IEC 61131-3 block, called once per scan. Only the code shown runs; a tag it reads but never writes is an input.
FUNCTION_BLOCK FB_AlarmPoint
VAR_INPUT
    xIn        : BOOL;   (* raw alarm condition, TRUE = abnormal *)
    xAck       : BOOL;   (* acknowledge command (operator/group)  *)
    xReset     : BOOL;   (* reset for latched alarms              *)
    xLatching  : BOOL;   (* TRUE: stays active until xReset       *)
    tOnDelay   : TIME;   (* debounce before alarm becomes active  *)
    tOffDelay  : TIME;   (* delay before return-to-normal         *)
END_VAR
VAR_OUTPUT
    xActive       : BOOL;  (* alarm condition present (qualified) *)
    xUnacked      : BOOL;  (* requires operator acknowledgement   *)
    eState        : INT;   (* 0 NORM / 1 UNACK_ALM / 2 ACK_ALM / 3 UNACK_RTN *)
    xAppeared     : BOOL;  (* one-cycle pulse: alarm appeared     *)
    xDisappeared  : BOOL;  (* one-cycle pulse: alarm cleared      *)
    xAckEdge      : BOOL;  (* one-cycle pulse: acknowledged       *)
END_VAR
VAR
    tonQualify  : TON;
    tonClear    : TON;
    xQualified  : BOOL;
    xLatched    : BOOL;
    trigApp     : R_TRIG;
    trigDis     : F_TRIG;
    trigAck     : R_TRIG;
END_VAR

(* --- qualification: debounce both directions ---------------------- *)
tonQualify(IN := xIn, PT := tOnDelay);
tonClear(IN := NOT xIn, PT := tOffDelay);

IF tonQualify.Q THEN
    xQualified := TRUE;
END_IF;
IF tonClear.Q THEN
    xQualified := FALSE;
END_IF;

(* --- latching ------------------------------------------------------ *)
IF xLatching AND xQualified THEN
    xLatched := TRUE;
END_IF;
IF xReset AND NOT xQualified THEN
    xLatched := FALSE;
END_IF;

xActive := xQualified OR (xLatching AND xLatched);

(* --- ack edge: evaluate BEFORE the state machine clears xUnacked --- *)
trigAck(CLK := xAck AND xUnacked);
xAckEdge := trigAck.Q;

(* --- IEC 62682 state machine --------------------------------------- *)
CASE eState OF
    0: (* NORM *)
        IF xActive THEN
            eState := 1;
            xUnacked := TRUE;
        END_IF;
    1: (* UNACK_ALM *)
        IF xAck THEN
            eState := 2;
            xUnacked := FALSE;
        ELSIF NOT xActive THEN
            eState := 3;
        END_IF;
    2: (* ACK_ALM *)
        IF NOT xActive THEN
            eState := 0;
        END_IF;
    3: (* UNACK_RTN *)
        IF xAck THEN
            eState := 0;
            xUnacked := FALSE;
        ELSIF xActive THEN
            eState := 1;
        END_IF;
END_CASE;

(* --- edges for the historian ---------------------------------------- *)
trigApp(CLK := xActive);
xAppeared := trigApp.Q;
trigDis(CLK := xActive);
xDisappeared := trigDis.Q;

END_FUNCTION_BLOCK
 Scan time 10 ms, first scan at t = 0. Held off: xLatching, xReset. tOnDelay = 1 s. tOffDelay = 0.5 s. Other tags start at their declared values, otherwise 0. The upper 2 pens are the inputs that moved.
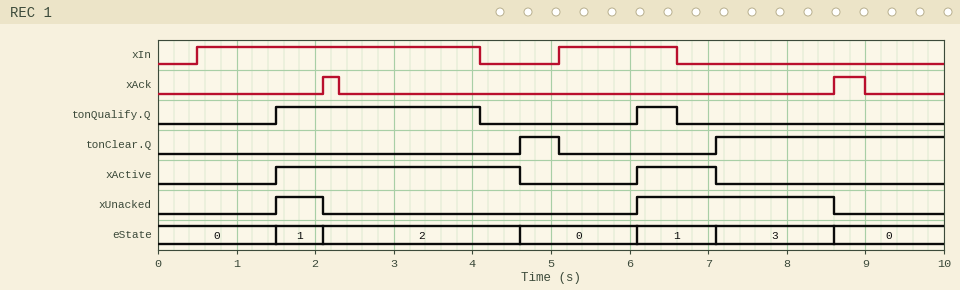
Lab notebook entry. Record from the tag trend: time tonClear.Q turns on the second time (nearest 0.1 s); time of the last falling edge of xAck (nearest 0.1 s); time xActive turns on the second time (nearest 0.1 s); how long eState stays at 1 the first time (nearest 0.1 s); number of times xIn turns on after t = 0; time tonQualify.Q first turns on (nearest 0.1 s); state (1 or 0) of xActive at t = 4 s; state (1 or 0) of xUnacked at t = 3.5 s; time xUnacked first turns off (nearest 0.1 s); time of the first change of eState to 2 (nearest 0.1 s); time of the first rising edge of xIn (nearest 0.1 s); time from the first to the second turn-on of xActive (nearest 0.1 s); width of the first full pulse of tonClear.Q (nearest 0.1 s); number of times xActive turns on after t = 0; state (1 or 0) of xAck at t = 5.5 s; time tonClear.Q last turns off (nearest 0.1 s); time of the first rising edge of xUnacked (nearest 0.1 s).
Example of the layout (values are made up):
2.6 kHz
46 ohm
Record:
7.1 s
9.0 s
6.1 s
0.6 s
2
1.5 s
1
0
2.1 s
2.1 s
0.5 s
4.6 s
0.5 s
2
0
5.1 s
1.5 s
